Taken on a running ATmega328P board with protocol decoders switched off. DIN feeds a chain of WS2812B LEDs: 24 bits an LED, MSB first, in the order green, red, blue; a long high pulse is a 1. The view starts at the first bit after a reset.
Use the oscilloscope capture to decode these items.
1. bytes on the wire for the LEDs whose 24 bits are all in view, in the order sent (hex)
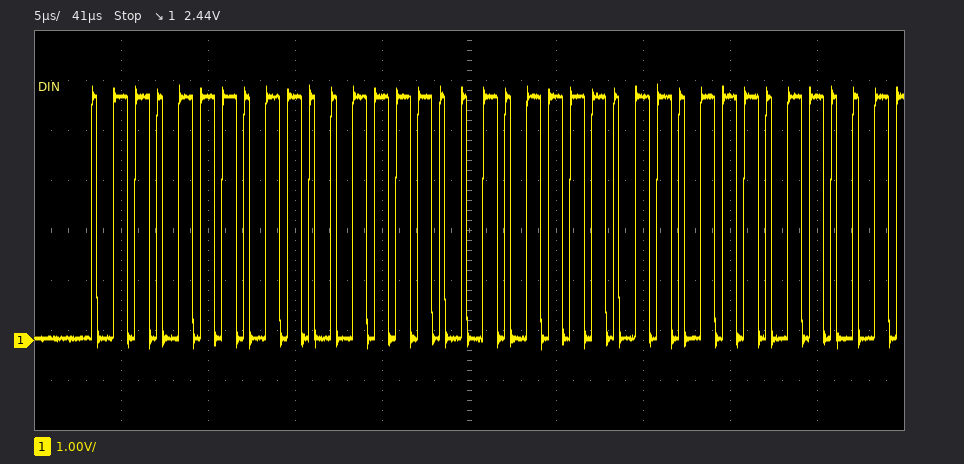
6E CF 2F
